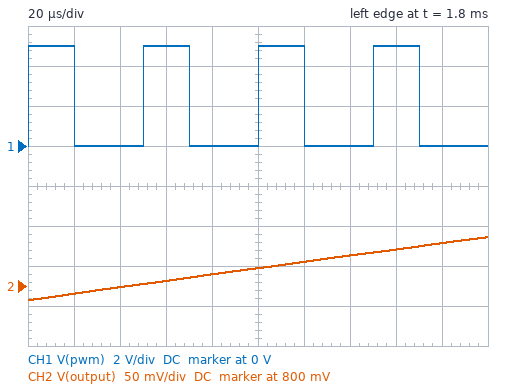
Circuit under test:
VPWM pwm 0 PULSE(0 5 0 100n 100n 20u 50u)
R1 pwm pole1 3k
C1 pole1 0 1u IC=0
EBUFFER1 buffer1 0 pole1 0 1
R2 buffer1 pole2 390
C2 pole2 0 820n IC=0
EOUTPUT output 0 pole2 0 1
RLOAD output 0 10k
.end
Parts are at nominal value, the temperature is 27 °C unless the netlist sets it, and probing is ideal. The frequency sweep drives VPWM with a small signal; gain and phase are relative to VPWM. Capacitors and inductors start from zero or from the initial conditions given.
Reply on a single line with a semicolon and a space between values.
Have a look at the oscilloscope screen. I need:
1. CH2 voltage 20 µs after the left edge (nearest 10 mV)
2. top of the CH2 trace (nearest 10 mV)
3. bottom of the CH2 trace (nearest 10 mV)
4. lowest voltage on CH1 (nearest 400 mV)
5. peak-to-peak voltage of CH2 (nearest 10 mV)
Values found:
790 mV; 860 mV; 780 mV; 0 V; 80 mV
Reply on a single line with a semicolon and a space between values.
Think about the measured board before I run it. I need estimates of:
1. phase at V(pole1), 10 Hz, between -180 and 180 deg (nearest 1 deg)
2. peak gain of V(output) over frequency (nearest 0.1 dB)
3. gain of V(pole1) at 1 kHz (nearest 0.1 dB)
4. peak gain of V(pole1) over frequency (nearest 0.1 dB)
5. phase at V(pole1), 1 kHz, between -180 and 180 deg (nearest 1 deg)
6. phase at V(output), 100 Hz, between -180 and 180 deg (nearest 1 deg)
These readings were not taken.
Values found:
-11 deg; 0 dB; -25.5 dB; 0 dB; -87 deg; -73 deg
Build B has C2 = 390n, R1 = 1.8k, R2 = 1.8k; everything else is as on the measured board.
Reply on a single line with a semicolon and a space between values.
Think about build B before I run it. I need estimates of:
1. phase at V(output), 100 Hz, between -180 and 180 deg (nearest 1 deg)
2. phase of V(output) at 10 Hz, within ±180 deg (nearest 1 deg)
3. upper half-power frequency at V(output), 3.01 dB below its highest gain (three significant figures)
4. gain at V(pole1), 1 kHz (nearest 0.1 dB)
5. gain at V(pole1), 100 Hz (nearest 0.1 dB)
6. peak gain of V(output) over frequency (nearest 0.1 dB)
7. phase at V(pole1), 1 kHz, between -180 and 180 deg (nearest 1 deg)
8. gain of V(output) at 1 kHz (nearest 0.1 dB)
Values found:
-72 deg; -9 deg; 78.4 Hz; -21.1 dB; -3.6 dB; 0 dB; -85 deg; -34.2 dB
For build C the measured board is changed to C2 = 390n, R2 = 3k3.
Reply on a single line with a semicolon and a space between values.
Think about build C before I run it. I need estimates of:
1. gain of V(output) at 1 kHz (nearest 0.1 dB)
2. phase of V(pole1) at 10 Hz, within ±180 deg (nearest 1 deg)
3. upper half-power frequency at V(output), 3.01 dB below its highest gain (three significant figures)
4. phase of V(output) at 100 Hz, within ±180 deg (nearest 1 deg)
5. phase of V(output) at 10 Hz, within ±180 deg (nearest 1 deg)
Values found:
-43.7 dB; -11 deg; 46.1 Hz; -101 deg; -15 deg
